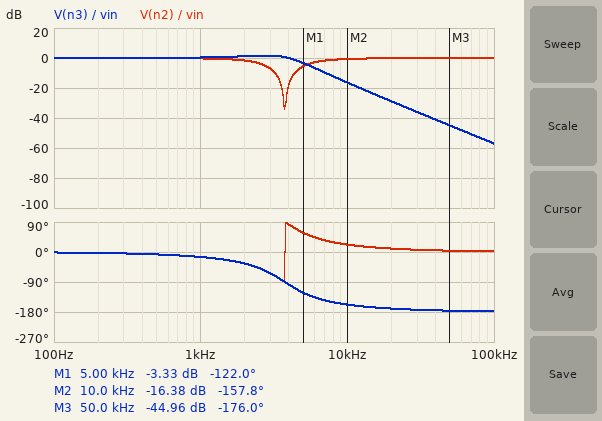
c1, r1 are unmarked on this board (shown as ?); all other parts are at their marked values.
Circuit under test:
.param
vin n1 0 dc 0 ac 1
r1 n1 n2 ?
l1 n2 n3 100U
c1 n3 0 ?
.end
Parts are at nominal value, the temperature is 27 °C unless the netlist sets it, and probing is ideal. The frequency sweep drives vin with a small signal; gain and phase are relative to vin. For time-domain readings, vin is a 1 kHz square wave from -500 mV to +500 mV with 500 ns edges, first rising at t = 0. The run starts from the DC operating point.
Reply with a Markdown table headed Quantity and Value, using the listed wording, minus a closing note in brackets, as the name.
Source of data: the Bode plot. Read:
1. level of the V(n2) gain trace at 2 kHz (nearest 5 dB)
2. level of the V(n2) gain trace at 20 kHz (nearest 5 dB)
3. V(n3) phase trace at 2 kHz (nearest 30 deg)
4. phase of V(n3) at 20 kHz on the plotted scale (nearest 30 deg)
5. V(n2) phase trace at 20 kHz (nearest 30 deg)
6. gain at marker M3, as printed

| Quantity | Value |
|---|---|
| level of the V(n2) gain trace at 2 kHz | 0 dB |
| level of the V(n2) gain trace at 20 kHz | 0 dB |
| V(n3) phase trace at 2 kHz | -30 deg |
| phase of V(n3) at 20 kHz on the plotted scale | -180 deg |
| V(n2) phase trace at 20 kHz | 0 deg |
| gain at marker M3, as printed | -44.96 dB |
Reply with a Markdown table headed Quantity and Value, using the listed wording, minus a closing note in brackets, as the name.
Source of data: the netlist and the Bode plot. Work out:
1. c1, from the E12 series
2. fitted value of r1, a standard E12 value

| Quantity | Value |
|---|---|
| c1, from the E12 series | 18 µF |
| fitted value of r1, a standard E12 value | 2.2 Ω |
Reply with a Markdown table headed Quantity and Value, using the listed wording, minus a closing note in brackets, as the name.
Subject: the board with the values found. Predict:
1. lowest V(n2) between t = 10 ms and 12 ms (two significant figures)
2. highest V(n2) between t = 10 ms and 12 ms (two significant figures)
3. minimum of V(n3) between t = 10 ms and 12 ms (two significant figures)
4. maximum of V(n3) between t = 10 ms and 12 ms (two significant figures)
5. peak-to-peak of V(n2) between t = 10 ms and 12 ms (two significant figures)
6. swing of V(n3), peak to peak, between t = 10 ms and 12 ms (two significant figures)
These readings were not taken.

| Quantity | Value |
|---|---|
| lowest V(n2) between t = 10 ms and 12 ms | -600 mV |
| highest V(n2) between t = 10 ms and 12 ms | 600 mV |
| minimum of V(n3) between t = 10 ms and 12 ms | -690 mV |
| maximum of V(n3) between t = 10 ms and 12 ms | 690 mV |
| peak-to-peak of V(n2) between t = 10 ms and 12 ms | 1.2 V |
| swing of V(n3), peak to peak, between t = 10 ms and 12 ms | 1.4 V |
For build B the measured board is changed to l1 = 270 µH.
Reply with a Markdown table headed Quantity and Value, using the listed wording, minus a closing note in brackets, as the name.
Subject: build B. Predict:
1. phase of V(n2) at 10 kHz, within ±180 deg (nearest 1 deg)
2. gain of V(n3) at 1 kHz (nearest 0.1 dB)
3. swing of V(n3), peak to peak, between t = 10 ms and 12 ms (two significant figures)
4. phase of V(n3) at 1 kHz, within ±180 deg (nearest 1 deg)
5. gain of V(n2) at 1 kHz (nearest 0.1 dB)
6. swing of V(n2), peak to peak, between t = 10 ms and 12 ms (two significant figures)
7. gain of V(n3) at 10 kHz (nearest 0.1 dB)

| Quantity | Value |
|---|---|
| phase of V(n2) at 10 kHz, within ±180 deg | 8 deg |
| gain of V(n3) at 1 kHz | 1.5 dB |
| swing of V(n3), peak to peak, between t = 10 ms and 12 ms | 1.7 V |
| phase of V(n3) at 1 kHz, within ±180 deg | -17 deg |
| gain of V(n2) at 1 kHz | -0.4 dB |
| swing of V(n2), peak to peak, between t = 10 ms and 12 ms | 1.3 V |
| gain of V(n3) at 10 kHz | -25.3 dB |
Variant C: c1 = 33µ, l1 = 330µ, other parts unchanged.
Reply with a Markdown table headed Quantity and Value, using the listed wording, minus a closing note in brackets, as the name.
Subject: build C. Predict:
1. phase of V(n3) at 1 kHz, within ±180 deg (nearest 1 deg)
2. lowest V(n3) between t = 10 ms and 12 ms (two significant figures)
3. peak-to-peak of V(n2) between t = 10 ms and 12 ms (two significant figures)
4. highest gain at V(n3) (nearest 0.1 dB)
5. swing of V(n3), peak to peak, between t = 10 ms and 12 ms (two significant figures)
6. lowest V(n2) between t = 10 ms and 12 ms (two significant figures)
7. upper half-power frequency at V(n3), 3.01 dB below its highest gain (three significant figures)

| Quantity | Value |
|---|---|
| phase of V(n3) at 1 kHz, within ±180 deg | -39 deg |
| lowest V(n3) between t = 10 ms and 12 ms | -840 mV |
| peak-to-peak of V(n2) between t = 10 ms and 12 ms | 1.3 V |
| highest gain at V(n3) | 3.7 dB |
| swing of V(n3), peak to peak, between t = 10 ms and 12 ms | 1.7 V |
| lowest V(n2) between t = 10 ms and 12 ms | -650 mV |
| upper half-power frequency at V(n3), 3.01 dB below its highest gain | 1.81 kHz |
